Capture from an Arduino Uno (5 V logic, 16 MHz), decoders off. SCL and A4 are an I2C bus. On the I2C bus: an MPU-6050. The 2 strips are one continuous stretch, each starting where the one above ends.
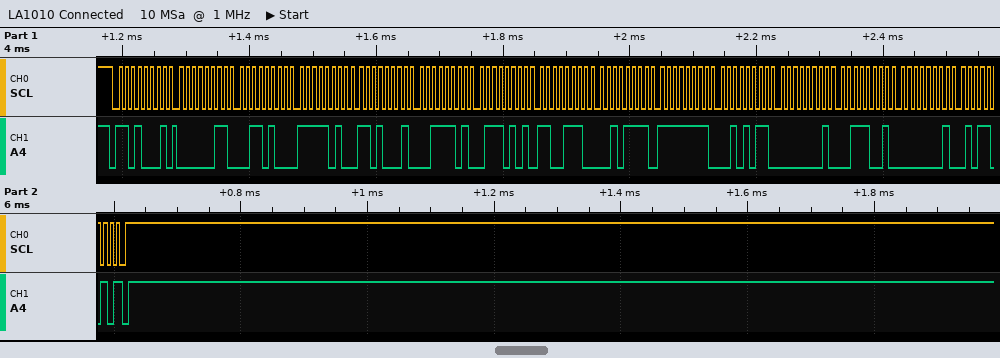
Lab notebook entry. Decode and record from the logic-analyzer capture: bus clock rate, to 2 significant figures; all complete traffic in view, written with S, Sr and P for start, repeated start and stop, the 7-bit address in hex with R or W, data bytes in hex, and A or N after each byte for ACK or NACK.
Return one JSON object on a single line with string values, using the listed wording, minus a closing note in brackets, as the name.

{"bus clock rate, to 2 significant figures": "100 kHz", "all complete traffic in view, written with S, Sr and P for start, repeated start and stop, the 7-bit address in hex with R or W, data bytes in hex, and A or N after each byte for ACK or NACK": "S 68R A 03 A 34 A FA A D1 A 3D A 75 A CE A 2F A FF A 2B A 01 A 39 A 01 A 5A N P"}
